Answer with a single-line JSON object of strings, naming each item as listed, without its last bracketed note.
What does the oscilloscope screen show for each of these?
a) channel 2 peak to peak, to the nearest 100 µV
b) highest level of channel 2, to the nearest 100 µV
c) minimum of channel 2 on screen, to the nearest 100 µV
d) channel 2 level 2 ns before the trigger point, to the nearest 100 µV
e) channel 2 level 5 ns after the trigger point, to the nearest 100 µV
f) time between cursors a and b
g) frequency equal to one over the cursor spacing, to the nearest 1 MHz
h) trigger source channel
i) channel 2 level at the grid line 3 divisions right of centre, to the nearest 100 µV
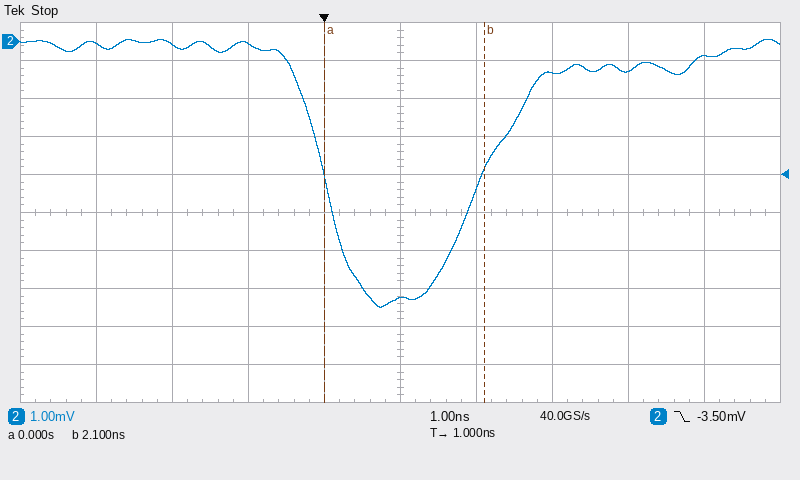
{"channel 2 peak to peak, to the nearest 100 µV": "7.1 mV", "highest level of channel 2, to the nearest 100 µV": "100 µV", "minimum of channel 2 on screen, to the nearest 100 µV": "-7.0 mV", "channel 2 level 2 ns before the trigger point, to the nearest 100 µV": "-100 µV", "channel 2 level 5 ns after the trigger point, to the nearest 100 µV": "-400 µV", "time between cursors a and b": "2.1 ns", "frequency equal to one over the cursor spacing, to the nearest 1 MHz": "476 MHz", "trigger source channel": "channel 2", "channel 2 level at the grid line 3 divisions right of centre, to the nearest 100 µV": "-800 µV"}
